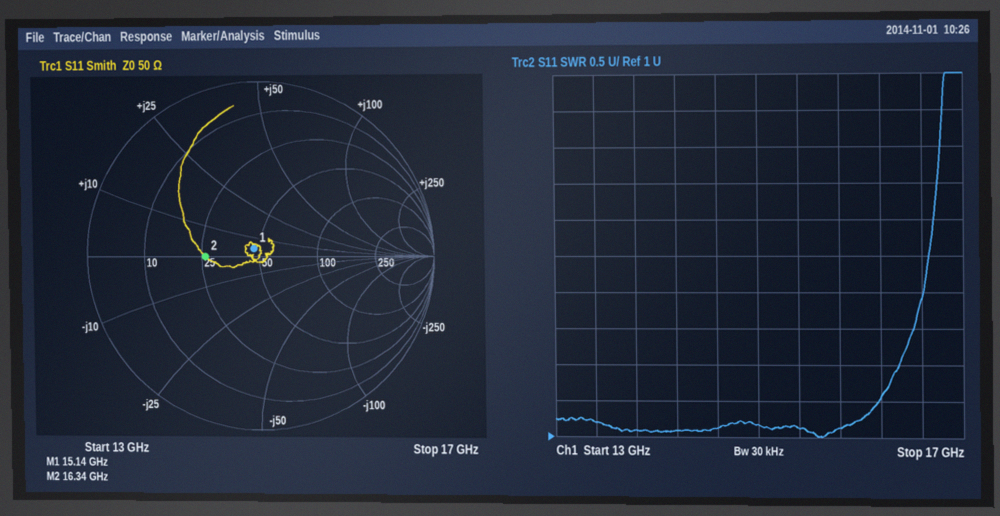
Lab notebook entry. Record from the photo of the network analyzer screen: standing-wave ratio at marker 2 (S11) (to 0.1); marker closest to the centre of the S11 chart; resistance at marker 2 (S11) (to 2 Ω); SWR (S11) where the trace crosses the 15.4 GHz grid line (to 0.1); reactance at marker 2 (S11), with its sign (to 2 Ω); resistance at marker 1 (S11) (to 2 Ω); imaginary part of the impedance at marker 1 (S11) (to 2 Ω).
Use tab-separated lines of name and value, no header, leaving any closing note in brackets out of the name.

standing-wave ratio at marker 2 (S11)	1.9
marker closest to the centre of the S11 chart	marker 1
resistance at marker 2 (S11)	26 Ω
SWR (S11) where the trace crosses the 15.4 GHz grid line	1.1
reactance at marker 2 (S11), with its sign	0 Ω
resistance at marker 1 (S11)	46 Ω
imaginary part of the impedance at marker 1 (S11)	+4 Ω
